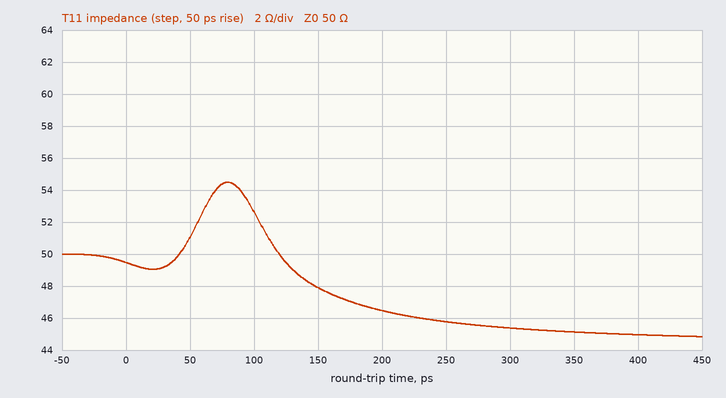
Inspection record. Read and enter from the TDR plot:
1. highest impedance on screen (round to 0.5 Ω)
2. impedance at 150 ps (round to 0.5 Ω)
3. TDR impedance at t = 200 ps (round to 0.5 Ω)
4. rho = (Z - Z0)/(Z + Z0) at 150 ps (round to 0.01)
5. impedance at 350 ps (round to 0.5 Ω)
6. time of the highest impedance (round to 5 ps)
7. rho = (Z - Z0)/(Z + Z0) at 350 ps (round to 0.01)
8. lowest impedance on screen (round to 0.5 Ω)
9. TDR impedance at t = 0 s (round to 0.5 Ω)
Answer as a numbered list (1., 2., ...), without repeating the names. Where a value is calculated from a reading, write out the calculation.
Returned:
1. 54.5 Ω
2. 48.0 Ω
3. 46.5 Ω
4. (48 − 50)/(48 + 50) ≈ -0.02
5. 45.0 Ω
6. 80 ps
7. (45 − 50)/(45 + 50) ≈ -0.05
8. 45.0 Ω
9. 49.5 Ω
